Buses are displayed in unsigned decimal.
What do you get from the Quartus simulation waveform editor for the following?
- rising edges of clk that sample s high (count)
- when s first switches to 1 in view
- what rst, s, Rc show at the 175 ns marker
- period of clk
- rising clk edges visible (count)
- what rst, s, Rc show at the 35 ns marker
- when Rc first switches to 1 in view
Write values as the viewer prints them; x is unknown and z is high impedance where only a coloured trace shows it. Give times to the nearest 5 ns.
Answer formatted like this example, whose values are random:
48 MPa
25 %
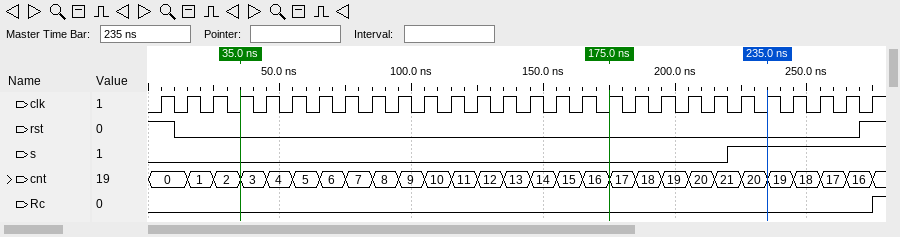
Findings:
6
220 ns
rst=0, s=0, Rc=0
10 ns
28
rst=0, s=0, Rc=0
275 ns
